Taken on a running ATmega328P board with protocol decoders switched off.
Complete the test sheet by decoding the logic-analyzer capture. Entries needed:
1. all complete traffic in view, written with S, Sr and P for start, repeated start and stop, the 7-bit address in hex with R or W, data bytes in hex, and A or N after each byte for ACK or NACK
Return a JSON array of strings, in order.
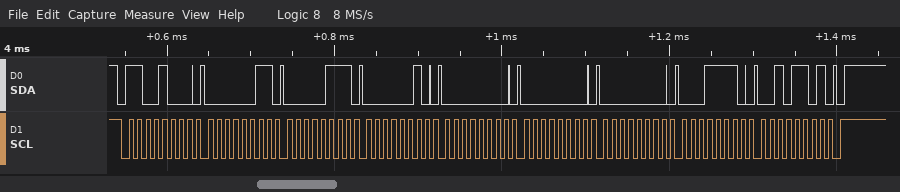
["S 64W A 03 A 07 A 02 A 00 A 00 A 00 A 1E A 2D A P"]
